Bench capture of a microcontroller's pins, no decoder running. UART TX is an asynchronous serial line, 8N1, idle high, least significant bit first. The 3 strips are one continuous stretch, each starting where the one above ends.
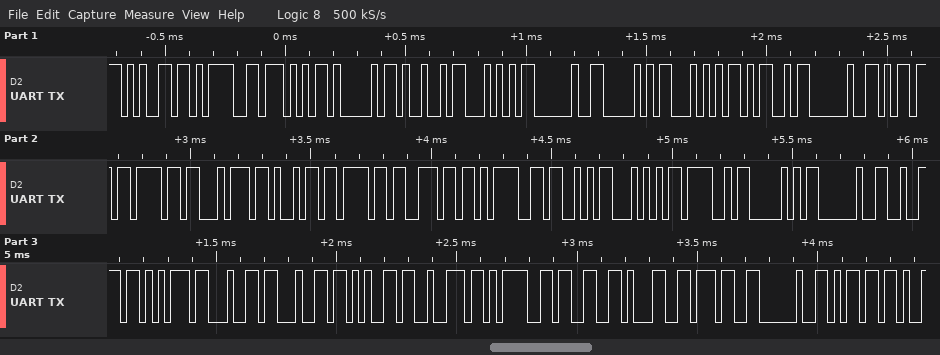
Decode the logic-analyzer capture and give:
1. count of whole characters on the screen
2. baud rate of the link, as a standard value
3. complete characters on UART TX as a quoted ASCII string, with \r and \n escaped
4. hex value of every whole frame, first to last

35
38400 baud
"e=WAIT PTM motion=STOP rudder=317 m"
0x65 0x3D 0x57 0x41 0x49 0x54 0x20 0x50 0x54 0x4D 0x20 0x6D 0x6F 0x74 0x69 0x6F 0x6E 0x3D 0x53 0x54 0x4F 0x50 0x20 0x72 0x75 0x64 0x64 0x65 0x72 0x3D 0x33 0x31 0x37 0x20 0x6D
